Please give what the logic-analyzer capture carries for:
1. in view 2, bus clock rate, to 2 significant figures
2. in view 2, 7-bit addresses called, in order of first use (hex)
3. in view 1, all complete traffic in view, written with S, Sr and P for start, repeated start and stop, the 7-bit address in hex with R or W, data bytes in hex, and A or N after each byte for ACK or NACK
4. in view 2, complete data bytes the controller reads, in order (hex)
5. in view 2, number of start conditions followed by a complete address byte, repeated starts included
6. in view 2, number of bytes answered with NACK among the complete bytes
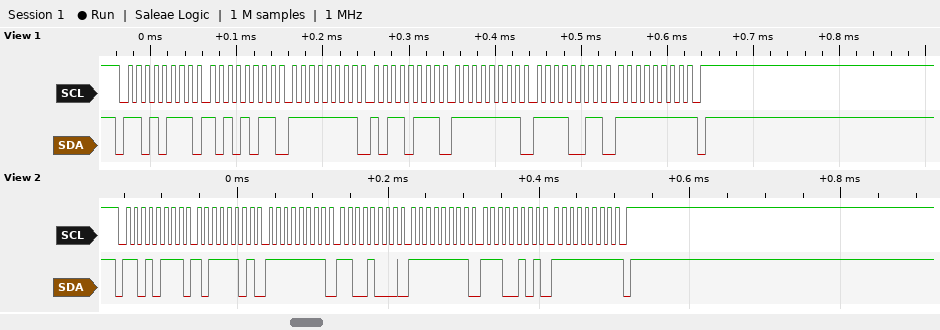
100 kHz
0x6B
S 6BR A AB A FF A B7 A FF A F3 A FF N P
BD FF C8 FF E5 FF
1
1
